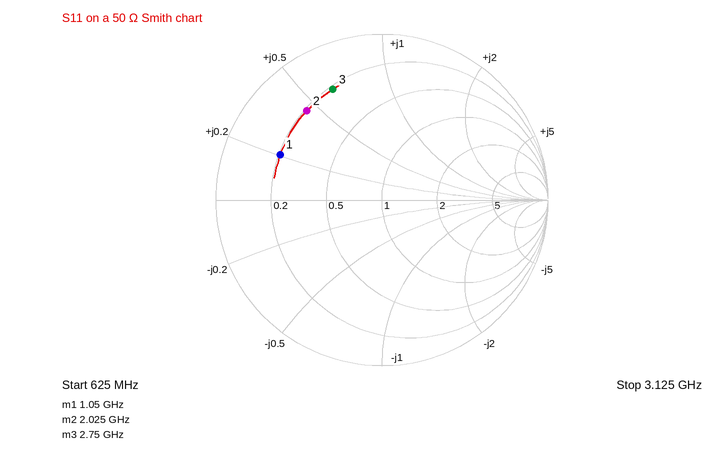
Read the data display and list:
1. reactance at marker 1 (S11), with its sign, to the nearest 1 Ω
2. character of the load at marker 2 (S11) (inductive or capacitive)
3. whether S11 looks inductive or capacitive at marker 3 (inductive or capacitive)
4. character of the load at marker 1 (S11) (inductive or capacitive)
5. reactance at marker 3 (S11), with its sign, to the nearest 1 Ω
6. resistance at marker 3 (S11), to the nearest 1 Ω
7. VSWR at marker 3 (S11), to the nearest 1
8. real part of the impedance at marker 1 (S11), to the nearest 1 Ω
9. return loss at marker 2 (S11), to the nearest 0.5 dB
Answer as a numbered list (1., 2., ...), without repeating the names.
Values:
1. +10 Ω
2. inductive
3. inductive
4. inductive
5. +31 Ω
6. 11 Ω
7. 6
8. 10 Ω
9. 3.0 dB
